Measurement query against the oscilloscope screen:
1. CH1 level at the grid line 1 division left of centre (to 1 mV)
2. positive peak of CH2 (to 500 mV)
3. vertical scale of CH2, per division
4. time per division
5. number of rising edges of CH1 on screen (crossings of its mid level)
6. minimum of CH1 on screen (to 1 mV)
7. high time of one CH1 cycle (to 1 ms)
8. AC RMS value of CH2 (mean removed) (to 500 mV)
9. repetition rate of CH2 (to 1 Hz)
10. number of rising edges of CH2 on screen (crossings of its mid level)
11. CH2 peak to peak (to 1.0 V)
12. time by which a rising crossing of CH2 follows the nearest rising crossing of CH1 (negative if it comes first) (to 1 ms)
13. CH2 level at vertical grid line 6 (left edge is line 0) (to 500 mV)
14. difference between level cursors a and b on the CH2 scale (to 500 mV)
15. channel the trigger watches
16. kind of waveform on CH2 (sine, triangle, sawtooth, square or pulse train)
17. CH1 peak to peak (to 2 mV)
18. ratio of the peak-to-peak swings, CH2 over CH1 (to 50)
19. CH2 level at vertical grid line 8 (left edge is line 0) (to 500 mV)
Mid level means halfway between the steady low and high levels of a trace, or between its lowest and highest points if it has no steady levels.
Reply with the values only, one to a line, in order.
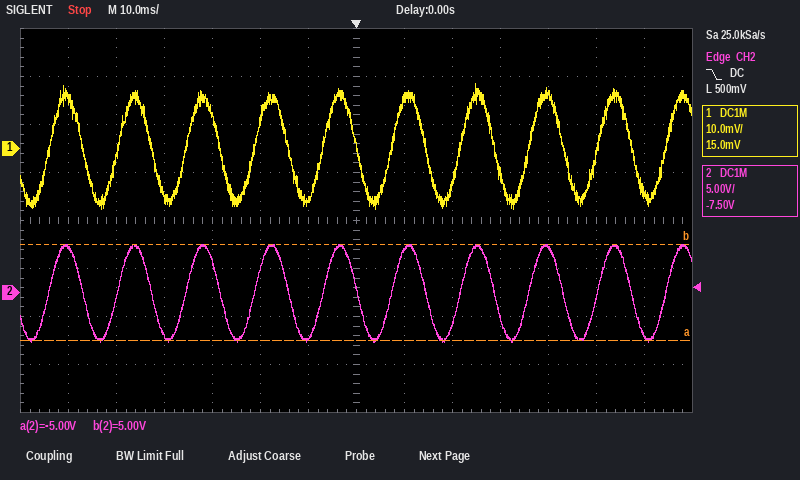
-11 mV
5.0 V
5 V
10 ms
10
-13 mV
7 ms
3.5 V
70 Hz
10
10.0 V
0 ms
-5.0 V
10.0 V
CH2
sine
26 mV
400
4.5 V
